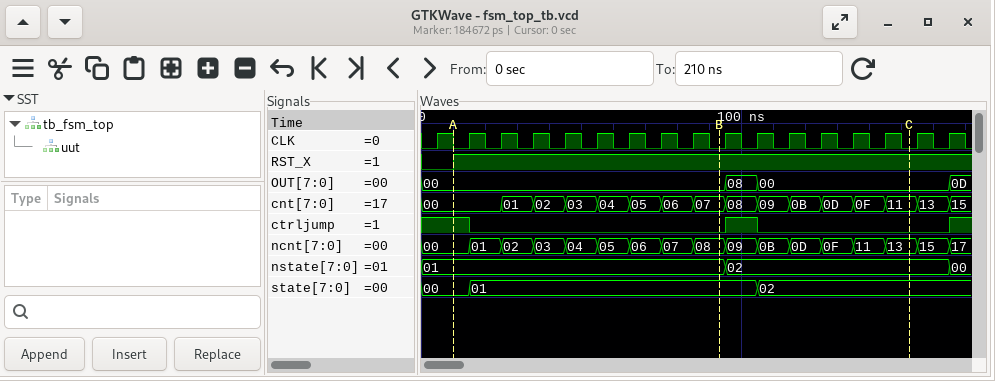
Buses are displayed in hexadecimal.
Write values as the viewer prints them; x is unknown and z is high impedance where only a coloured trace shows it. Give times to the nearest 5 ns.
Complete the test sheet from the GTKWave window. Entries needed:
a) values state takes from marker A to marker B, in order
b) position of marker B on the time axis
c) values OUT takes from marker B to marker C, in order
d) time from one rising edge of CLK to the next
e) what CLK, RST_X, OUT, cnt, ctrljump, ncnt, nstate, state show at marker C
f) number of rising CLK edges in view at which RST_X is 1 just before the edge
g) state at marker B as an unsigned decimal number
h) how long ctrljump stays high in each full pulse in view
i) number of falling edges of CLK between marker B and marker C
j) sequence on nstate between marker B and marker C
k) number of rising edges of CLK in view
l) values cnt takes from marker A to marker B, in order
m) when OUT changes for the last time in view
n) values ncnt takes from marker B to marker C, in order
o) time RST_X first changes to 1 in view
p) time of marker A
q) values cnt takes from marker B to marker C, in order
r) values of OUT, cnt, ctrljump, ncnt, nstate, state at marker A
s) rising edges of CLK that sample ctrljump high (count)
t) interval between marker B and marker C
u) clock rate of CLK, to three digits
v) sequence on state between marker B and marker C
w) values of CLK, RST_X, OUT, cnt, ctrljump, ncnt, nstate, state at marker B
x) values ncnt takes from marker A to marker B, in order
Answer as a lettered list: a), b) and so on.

a) 00, 01
b) 95 ns
c) 00, 08, 00
d) 10 ns
e) CLK=0, RST_X=1, OUT=00, cnt=11, ctrljump=0, ncnt=13, nstate=02, state=02
f) 16
g) 1
h) 10 ns
i) 6
j) 01, 02
k) 17
l) 00, 01, 02, 03, 04, 05, 06, 07
m) 165 ns
n) 08, 09, 0B, 0D, 0F, 11, 13
o) 10 ns
p) 10 ns
q) 07, 08, 09, 0B, 0D, 0F, 11
r) OUT=00, cnt=00, ctrljump=1, ncnt=00, nstate=01, state=00
s) 3
t) 60 ns
u) 100 MHz
v) 01, 02
w) CLK=0, RST_X=1, OUT=00, cnt=07, ctrljump=0, ncnt=08, nstate=01, state=01
x) 00, 01, 02, 03, 04, 05, 06, 07, 08
